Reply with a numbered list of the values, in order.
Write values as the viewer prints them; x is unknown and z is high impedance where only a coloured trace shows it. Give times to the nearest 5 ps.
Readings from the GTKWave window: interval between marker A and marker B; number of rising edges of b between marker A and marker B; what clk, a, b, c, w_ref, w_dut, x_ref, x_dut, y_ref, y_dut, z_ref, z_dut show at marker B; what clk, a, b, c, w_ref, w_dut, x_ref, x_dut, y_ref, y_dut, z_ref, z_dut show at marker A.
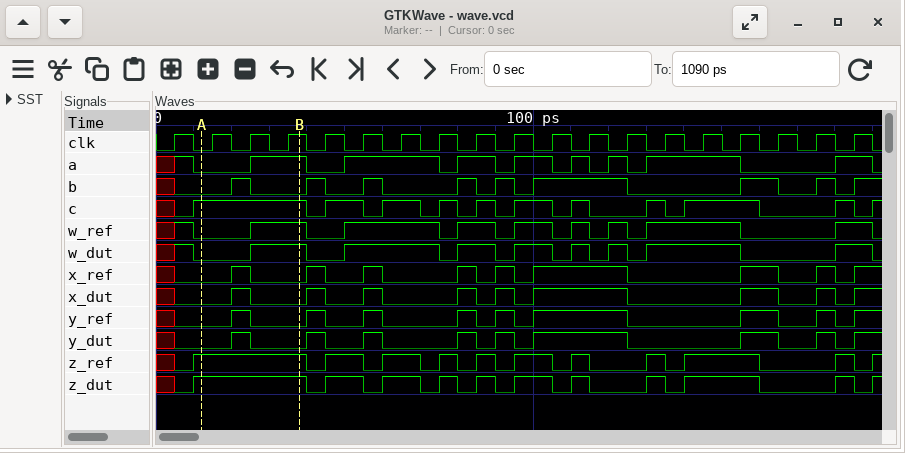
1. 25 ps
2. 1
3. clk=1, a=1, b=0, c=1, w_ref=1, w_dut=1, x_ref=0, x_dut=0, y_ref=0, y_dut=0, z_ref=1, z_dut=1
4. clk=0, a=0, b=0, c=1, w_ref=0, w_dut=0, x_ref=0, x_dut=0, y_ref=0, y_dut=0, z_ref=1, z_dut=1
